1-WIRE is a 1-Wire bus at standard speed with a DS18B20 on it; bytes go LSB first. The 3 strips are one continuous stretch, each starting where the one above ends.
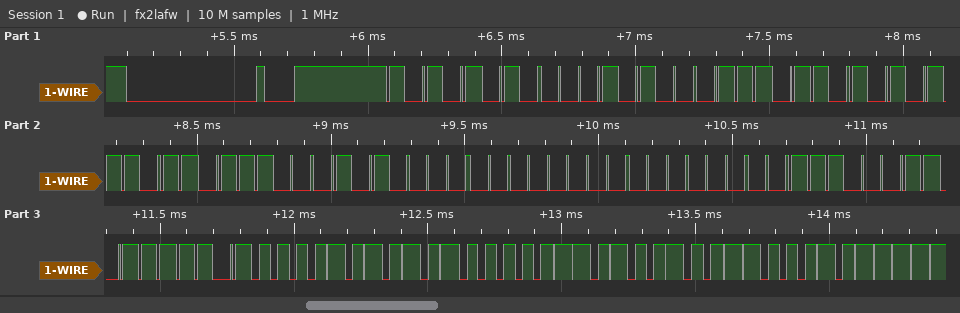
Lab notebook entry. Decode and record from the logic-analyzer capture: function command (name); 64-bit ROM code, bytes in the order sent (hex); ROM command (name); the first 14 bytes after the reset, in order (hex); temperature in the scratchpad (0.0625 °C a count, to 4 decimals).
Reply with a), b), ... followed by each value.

a) Read Scratchpad
b) 28 6E 75 3B 0A 00 00 C7
c) Match ROM
d) 55 28 6E 75 3B 0A 00 00 C7 BE 50 05 4B 46
e) 85.0000 °C
